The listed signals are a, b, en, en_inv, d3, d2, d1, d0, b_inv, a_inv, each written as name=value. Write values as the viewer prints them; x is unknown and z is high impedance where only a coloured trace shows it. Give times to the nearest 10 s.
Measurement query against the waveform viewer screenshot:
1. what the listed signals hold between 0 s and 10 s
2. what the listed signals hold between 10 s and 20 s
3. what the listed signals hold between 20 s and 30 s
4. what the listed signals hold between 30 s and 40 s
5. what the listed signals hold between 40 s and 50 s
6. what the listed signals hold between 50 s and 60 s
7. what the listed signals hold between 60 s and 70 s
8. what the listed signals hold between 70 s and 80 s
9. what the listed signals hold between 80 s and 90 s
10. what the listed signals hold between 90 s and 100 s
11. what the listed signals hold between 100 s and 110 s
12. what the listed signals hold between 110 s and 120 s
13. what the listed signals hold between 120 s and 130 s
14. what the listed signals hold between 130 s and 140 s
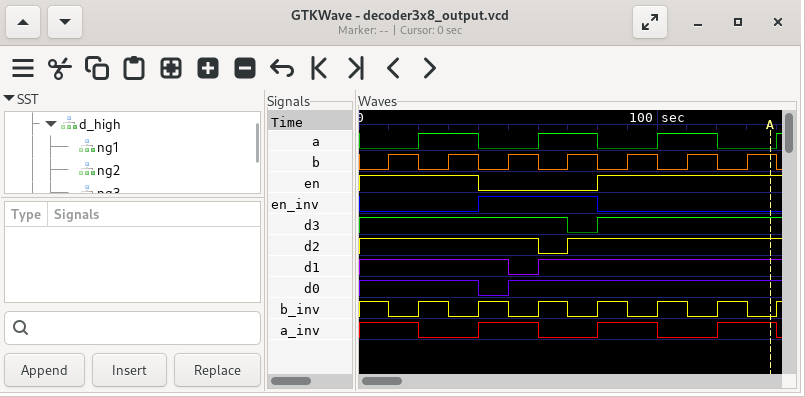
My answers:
a=0, b=0, en=1, en_inv=0, d3=1, d2=1, d1=1, d0=1, b_inv=1, a_inv=1
a=0, b=1, en=1, en_inv=0, d3=1, d2=1, d1=1, d0=1, b_inv=0, a_inv=1
a=1, b=0, en=1, en_inv=0, d3=1, d2=1, d1=1, d0=1, b_inv=1, a_inv=0
a=1, b=1, en=1, en_inv=0, d3=1, d2=1, d1=1, d0=1, b_inv=0, a_inv=0
a=0, b=0, en=0, en_inv=1, d3=1, d2=1, d1=1, d0=0, b_inv=1, a_inv=1
a=0, b=1, en=0, en_inv=1, d3=1, d2=1, d1=0, d0=1, b_inv=0, a_inv=1
a=1, b=0, en=0, en_inv=1, d3=1, d2=0, d1=1, d0=1, b_inv=1, a_inv=0
a=1, b=1, en=0, en_inv=1, d3=0, d2=1, d1=1, d0=1, b_inv=0, a_inv=0
a=0, b=0, en=1, en_inv=0, d3=1, d2=1, d1=1, d0=1, b_inv=1, a_inv=1
a=0, b=1, en=1, en_inv=0, d3=1, d2=1, d1=1, d0=1, b_inv=0, a_inv=1
a=1, b=0, en=1, en_inv=0, d3=1, d2=1, d1=1, d0=1, b_inv=1, a_inv=0
a=1, b=1, en=1, en_inv=0, d3=1, d2=1, d1=1, d0=1, b_inv=0, a_inv=0
a=0, b=0, en=1, en_inv=0, d3=1, d2=1, d1=1, d0=1, b_inv=1, a_inv=1
a=0, b=1, en=1, en_inv=0, d3=1, d2=1, d1=1, d0=1, b_inv=0, a_inv=1
